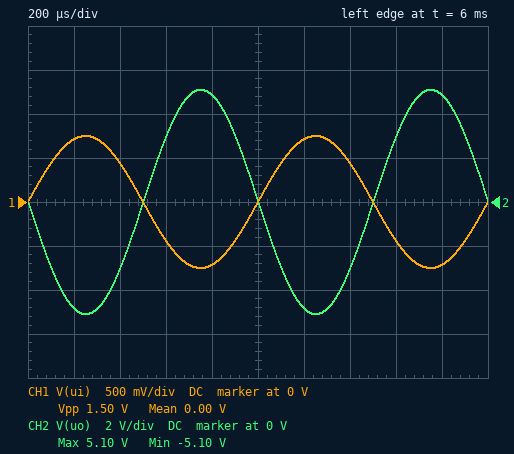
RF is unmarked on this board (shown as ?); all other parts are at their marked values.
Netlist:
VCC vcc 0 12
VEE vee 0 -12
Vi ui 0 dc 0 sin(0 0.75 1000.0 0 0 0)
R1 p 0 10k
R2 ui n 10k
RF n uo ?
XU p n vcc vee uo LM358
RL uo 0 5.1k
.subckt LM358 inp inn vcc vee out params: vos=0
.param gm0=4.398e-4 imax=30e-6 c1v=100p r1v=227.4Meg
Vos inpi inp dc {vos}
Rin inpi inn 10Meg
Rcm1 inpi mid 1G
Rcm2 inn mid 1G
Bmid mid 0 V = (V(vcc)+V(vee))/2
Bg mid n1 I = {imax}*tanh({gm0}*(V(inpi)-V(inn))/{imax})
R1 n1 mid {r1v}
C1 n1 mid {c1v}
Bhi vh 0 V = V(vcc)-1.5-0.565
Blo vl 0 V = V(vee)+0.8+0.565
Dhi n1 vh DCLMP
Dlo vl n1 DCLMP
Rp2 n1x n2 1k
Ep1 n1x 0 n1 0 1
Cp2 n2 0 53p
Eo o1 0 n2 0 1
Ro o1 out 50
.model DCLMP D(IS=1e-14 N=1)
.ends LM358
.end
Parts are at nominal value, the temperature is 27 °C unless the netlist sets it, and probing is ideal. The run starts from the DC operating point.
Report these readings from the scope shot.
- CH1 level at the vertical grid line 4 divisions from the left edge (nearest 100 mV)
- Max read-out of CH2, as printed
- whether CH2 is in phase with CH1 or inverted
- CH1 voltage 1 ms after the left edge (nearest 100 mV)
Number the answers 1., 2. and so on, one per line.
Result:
1. -700 mV
2. 5.10 V
3. inverted
4. 0 V
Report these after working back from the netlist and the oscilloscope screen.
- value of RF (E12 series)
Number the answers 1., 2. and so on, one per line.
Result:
1. 68 kΩ
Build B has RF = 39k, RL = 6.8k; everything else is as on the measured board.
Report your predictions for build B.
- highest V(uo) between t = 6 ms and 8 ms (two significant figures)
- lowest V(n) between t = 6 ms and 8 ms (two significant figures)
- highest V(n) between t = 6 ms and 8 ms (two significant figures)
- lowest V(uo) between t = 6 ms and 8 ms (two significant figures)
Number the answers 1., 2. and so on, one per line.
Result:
1. 2.9 V
2. -4.2 mV
3. 4.2 mV
4. -2.9 V
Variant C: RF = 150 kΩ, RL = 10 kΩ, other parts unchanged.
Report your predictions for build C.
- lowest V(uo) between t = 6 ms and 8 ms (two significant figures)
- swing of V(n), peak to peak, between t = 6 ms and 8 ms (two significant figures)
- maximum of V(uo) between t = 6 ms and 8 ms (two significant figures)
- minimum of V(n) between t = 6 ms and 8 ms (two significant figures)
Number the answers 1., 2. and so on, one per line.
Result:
1. -11 V
2. 68 mV
3. 10 V
4. -51 mV
